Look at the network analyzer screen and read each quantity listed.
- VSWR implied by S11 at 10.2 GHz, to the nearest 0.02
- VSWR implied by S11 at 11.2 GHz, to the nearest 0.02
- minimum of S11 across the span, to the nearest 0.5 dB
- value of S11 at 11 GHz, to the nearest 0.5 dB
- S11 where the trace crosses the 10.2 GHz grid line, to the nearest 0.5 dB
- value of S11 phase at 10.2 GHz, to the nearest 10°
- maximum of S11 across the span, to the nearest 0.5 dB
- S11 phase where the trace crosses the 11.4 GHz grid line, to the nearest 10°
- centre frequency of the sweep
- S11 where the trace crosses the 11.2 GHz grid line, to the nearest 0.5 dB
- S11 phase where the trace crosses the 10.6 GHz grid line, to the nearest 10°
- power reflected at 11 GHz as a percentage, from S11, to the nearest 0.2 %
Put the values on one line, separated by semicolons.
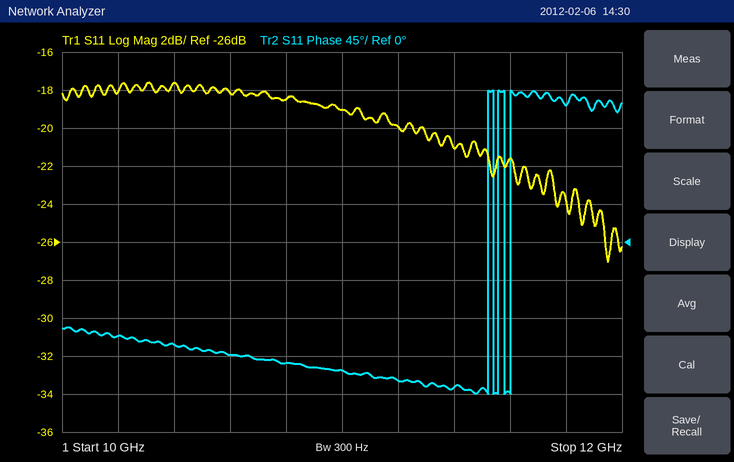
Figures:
1.28; 1.22; -27.0 dB; -19.0 dB; -18.0 dB; -110°; -17.5 dB; -170°; 11 GHz; -20.0 dB; -130°; 1.2 %
